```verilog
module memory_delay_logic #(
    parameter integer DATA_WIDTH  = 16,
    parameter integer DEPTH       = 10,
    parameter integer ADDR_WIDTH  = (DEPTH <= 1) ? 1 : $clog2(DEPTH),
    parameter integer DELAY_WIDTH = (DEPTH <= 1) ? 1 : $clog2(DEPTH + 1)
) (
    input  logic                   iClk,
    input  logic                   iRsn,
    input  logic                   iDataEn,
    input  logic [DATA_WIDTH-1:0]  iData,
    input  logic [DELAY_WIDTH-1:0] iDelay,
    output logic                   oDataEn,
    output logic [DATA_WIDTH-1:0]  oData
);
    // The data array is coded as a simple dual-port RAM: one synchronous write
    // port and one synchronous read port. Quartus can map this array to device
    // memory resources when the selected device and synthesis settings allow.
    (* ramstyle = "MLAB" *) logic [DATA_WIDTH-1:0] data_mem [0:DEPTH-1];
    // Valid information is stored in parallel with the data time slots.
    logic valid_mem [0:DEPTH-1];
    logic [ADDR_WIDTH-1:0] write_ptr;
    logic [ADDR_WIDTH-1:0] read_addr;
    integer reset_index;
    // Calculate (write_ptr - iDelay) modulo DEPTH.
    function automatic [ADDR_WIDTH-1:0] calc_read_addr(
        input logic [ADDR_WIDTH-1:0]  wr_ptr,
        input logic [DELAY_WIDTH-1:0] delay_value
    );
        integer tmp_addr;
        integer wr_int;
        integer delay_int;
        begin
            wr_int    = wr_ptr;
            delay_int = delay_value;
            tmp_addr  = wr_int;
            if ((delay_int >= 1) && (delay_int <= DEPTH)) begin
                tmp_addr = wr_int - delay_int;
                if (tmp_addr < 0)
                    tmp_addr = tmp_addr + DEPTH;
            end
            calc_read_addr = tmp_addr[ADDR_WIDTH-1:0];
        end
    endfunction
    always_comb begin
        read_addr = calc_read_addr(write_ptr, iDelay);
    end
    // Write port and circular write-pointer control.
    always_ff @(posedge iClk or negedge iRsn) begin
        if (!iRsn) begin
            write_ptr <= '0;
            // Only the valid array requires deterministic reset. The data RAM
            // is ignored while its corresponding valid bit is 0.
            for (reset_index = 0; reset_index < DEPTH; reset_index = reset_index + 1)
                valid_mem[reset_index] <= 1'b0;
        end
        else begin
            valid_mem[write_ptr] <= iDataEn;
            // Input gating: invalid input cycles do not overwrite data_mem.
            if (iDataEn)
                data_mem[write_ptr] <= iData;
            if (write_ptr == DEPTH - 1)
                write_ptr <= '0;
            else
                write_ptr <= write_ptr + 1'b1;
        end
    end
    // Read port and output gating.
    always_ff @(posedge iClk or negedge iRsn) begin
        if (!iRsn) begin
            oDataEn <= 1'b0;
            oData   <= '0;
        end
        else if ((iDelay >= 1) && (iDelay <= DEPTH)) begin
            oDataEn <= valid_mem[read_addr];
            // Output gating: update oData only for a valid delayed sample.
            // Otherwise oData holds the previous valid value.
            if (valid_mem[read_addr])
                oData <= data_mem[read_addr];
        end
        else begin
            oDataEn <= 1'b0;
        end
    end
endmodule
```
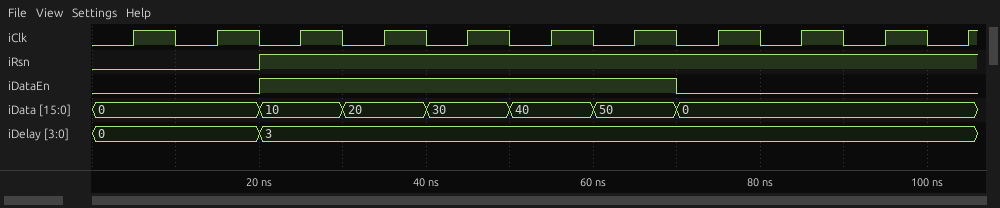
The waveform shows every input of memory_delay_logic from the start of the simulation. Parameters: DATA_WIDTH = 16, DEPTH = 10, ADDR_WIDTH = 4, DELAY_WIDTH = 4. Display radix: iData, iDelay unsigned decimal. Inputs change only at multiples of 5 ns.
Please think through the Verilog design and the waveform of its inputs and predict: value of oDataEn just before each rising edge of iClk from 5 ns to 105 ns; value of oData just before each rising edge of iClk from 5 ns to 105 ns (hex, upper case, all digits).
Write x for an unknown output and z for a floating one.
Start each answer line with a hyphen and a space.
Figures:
- 0 0 0 0 0 0 1 1 1 1 1
- 0000, 0000, 0000, 0000, 0000, 0000, 000A, 0014, 001E, 0028, 0032
